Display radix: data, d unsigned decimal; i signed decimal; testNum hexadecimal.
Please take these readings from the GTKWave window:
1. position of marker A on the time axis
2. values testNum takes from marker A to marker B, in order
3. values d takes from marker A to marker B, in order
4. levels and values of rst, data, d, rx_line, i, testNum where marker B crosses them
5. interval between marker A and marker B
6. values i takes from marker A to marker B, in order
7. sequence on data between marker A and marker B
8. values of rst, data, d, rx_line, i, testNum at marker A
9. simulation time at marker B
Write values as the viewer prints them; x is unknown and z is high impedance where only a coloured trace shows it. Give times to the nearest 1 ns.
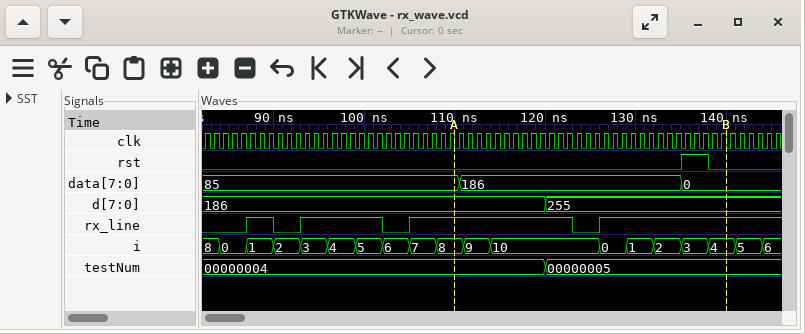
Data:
110 ns
00000004, 00000005
186, 255
rst=0, data=0, d=255, rx_line=1, i=4, testNum=00000005
30 ns
8, 9, 10, 0, 1, 2, 3, 4
85, 186, 0
rst=0, data=85, d=186, rx_line=1, i=8, testNum=00000004
140 ns
